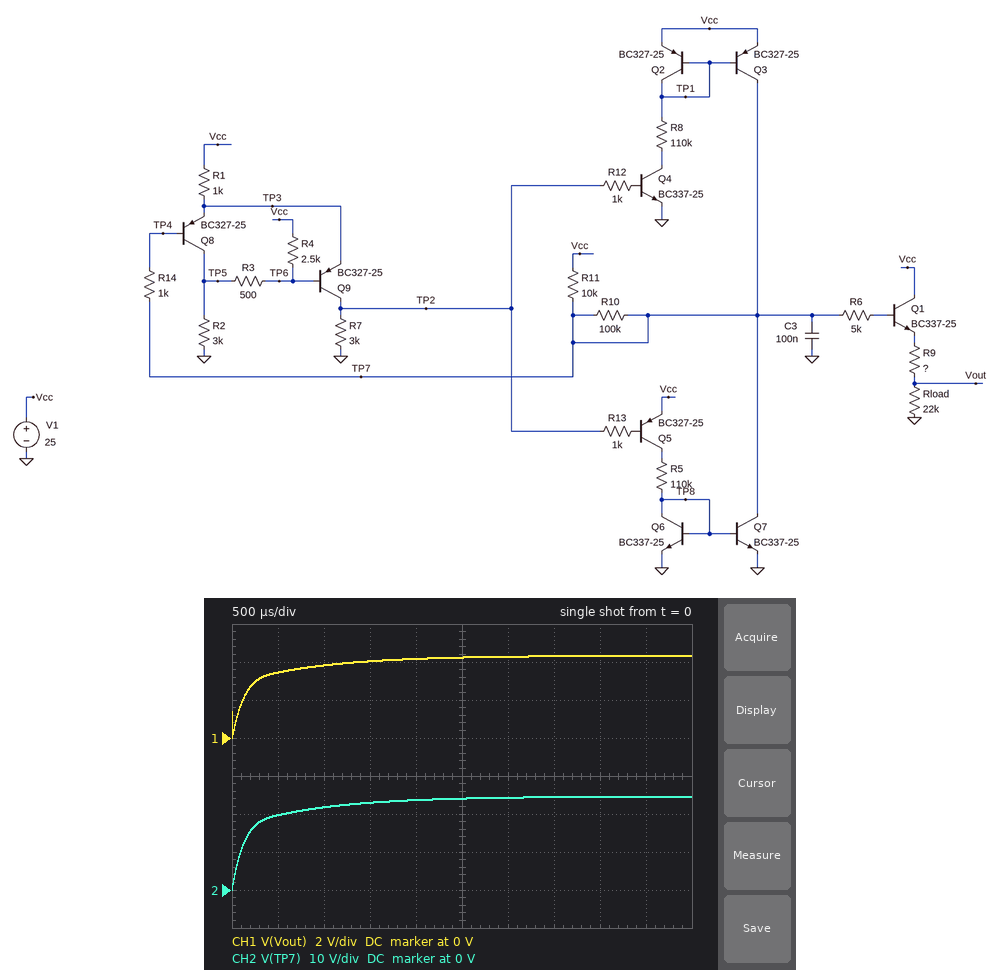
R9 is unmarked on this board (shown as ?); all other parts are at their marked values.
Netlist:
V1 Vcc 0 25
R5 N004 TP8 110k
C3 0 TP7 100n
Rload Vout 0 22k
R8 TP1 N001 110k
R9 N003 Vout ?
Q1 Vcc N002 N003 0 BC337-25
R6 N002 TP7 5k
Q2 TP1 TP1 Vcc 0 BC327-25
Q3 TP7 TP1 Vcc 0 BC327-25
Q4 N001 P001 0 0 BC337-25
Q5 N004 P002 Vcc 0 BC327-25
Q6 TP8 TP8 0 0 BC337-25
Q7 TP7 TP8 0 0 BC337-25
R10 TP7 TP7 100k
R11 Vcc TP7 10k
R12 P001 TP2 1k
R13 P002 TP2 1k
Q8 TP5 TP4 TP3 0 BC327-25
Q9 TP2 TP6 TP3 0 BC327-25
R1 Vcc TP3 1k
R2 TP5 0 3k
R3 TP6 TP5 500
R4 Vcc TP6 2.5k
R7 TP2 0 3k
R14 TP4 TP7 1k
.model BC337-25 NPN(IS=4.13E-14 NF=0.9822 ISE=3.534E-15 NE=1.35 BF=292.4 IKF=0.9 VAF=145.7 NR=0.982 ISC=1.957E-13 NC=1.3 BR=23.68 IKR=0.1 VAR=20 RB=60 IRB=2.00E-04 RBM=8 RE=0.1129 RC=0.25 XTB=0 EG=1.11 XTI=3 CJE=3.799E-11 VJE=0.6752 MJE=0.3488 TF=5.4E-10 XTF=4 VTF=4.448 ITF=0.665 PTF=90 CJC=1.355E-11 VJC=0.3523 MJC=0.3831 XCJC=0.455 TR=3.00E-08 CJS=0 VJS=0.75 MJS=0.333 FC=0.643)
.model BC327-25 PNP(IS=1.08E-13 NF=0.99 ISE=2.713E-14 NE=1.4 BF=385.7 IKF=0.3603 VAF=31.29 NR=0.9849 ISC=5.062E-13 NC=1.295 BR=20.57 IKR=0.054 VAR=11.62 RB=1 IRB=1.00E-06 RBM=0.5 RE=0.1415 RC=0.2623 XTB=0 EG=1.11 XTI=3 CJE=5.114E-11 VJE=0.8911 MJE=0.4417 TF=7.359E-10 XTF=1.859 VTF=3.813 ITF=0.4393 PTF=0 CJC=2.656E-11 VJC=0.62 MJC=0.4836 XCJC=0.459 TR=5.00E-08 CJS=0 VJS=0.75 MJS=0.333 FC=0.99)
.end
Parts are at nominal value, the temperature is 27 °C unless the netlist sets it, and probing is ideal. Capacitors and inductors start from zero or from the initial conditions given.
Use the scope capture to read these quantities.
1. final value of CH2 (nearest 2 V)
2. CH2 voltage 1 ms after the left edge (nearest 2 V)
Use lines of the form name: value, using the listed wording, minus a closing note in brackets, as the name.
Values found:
final value of CH2: 24 V
CH2 voltage 1 ms after the left edge: 22 V
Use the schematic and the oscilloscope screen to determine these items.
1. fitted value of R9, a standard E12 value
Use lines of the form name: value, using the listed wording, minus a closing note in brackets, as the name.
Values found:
fitted value of R9, a standard E12 value: 100 kΩ
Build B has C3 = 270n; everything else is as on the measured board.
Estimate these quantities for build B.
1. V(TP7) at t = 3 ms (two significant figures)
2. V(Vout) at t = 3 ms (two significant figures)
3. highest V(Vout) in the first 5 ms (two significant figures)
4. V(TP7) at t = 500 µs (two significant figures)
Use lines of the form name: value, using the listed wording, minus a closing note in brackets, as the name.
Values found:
V(TP7) at t = 3 ms: 22 V
V(Vout) at t = 3 ms: 3.9 V
highest V(Vout) in the first 5 ms: 4.1 V
V(TP7) at t = 500 µs: 15 V
